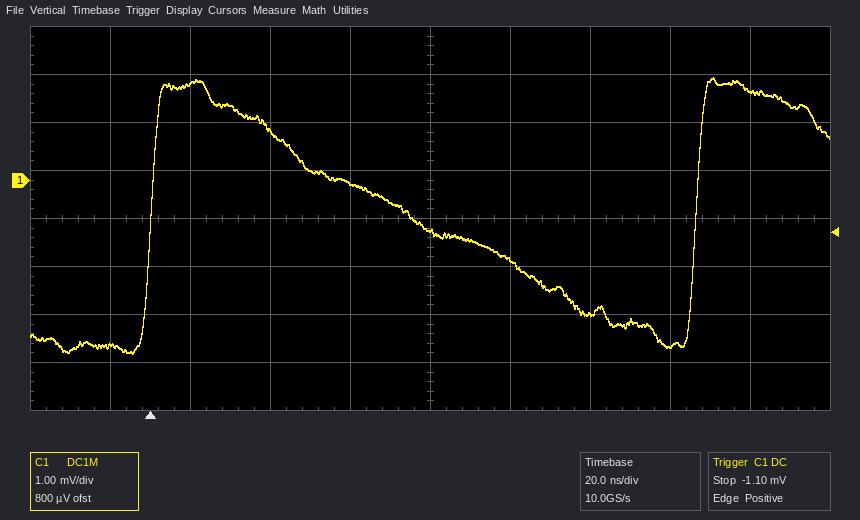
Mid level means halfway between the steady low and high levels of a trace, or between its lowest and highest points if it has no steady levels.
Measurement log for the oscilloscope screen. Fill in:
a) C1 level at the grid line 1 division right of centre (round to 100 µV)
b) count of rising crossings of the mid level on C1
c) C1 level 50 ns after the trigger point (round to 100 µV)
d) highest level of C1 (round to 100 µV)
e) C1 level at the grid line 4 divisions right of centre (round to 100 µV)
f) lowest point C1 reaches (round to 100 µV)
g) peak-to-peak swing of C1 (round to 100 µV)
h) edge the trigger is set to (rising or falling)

-1.7 mV
2
-100 µV
2.1 mV
1.9 mV
-3.6 mV
5.7 mV
rising
